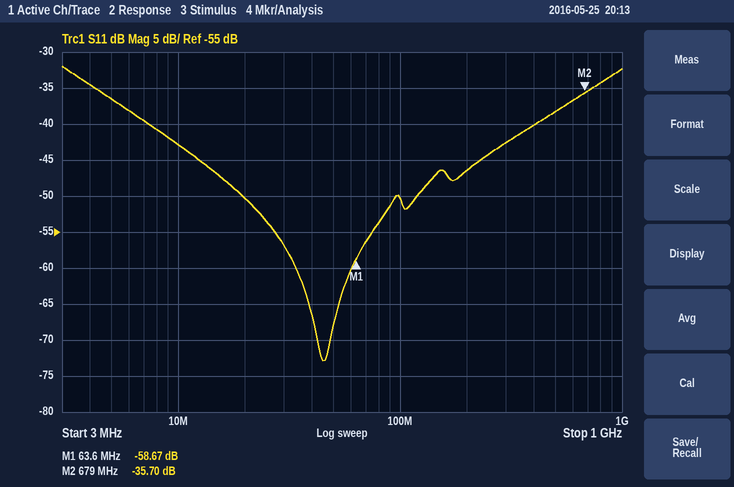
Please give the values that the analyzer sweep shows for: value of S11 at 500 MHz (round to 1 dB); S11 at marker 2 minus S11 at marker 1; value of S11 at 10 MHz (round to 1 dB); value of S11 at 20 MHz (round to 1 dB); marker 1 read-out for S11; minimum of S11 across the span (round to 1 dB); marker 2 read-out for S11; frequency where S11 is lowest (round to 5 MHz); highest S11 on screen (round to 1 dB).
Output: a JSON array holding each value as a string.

["-38 dB", "22.97 dB", "-43 dB", "-50 dB", "-58.67 dB", "-73 dB", "-35.70 dB", "45 MHz", "-32 dB"]
